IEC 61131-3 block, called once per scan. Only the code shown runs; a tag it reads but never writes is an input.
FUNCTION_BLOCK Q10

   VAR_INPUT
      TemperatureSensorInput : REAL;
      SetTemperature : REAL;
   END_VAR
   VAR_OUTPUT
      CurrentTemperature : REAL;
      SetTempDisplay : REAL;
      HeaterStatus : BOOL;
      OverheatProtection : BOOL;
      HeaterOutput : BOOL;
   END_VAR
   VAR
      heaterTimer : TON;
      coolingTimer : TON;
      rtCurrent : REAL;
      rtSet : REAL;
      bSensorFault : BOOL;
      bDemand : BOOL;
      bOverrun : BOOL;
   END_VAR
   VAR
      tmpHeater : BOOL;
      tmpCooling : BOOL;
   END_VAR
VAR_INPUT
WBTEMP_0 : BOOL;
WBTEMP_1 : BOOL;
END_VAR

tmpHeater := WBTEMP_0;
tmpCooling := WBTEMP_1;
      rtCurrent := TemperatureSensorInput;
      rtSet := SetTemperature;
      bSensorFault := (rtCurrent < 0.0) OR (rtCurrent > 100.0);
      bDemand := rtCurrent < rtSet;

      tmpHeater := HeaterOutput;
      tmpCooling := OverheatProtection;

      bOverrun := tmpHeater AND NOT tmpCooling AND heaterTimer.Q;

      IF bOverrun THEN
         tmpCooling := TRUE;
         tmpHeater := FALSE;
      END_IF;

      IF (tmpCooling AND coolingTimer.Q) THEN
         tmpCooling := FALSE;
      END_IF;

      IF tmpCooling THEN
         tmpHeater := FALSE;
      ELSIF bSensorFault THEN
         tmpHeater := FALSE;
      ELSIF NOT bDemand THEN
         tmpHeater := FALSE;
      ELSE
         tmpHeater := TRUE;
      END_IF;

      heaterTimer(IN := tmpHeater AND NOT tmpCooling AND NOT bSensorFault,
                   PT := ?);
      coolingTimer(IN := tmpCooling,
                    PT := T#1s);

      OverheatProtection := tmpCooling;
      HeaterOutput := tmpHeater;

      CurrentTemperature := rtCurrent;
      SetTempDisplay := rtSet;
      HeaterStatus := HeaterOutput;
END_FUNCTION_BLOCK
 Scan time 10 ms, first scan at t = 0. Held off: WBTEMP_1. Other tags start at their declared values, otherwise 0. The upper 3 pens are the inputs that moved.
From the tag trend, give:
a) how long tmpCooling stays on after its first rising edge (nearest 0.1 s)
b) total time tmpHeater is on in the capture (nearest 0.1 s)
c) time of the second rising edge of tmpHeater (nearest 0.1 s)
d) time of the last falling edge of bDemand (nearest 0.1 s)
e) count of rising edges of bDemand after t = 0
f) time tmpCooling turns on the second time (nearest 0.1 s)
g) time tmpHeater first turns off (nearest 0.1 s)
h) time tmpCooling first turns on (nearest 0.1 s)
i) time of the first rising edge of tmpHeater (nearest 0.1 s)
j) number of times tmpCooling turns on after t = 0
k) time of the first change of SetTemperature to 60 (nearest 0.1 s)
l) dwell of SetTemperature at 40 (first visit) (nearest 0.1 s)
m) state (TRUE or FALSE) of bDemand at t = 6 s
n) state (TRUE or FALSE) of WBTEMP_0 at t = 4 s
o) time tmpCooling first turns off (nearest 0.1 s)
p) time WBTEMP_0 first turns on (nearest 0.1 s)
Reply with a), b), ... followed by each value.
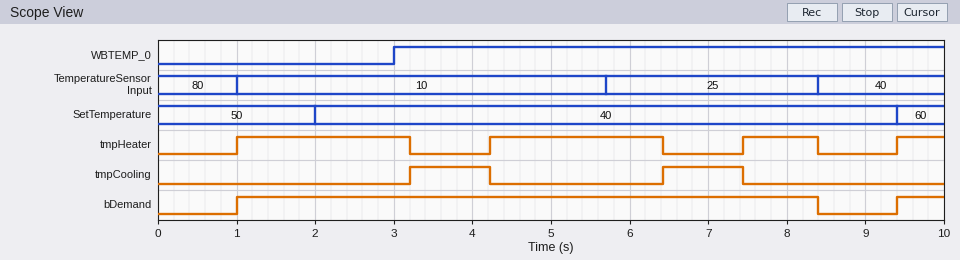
a) 1.0 s
b) 6.0 s
c) 4.2 s
d) 8.4 s
e) 2
f) 6.4 s
g) 3.2 s
h) 3.2 s
i) 1.0 s
j) 2
k) 9.4 s
l) 7.4 s
m) TRUE
n) TRUE
o) 4.2 s
p) 3.0 s
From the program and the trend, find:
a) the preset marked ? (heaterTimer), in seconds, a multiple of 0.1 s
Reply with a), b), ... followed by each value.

a) 2.2 s
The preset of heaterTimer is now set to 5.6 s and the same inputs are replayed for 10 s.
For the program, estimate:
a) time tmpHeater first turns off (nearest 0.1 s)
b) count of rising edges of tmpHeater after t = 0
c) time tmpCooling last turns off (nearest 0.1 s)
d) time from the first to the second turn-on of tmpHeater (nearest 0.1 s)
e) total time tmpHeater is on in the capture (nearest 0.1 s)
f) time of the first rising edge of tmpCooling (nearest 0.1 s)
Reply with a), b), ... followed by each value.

a) 6.6 s
b) 3
c) 7.6 s
d) 6.6 s
e) 7.0 s
f) 6.6 s
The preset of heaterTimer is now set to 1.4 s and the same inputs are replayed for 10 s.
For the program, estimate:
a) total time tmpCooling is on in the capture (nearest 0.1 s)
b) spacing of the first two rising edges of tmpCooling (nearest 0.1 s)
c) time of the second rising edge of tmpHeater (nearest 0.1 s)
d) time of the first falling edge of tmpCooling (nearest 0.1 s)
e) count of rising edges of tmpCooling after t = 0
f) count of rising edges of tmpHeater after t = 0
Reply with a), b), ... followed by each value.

a) 3.0 s
b) 2.4 s
c) 3.4 s
d) 3.4 s
e) 3
f) 5
